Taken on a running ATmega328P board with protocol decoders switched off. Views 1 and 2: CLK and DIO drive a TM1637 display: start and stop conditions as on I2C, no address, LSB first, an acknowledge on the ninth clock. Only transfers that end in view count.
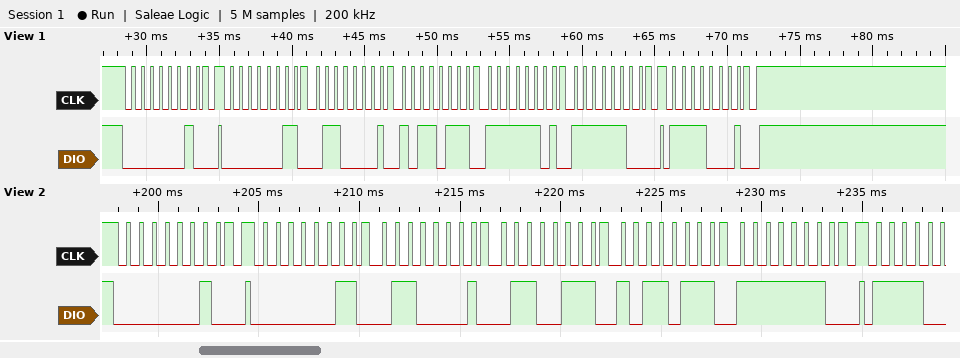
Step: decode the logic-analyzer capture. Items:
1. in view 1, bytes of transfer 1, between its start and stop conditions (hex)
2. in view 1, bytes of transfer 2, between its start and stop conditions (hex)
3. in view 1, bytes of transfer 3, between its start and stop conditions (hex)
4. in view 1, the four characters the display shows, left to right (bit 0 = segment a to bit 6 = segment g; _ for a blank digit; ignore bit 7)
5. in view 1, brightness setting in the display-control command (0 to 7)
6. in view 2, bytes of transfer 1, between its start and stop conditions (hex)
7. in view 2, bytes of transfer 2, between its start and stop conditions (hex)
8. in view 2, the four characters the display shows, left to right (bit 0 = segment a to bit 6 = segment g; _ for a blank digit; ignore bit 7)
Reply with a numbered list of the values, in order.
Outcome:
1. 40
2. C0 86 ED BF 3F
3. 8F
4. 1500
5. 7
6. 40
7. C0 86 E6 ED 7F
8. 1458
